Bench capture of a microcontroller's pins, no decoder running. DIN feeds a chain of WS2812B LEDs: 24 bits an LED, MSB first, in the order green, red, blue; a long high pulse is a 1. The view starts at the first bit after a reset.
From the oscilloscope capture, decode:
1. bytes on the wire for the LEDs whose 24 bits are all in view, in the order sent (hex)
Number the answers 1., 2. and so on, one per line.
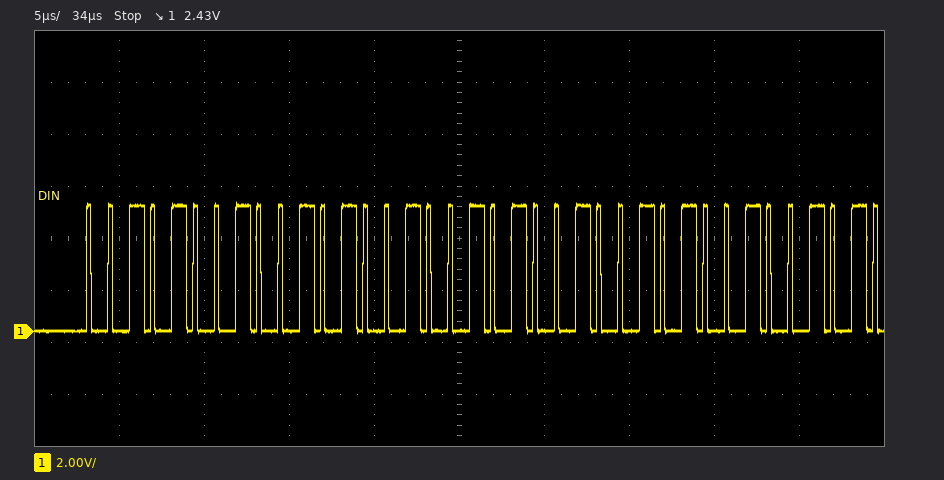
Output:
1. 29 29 29
